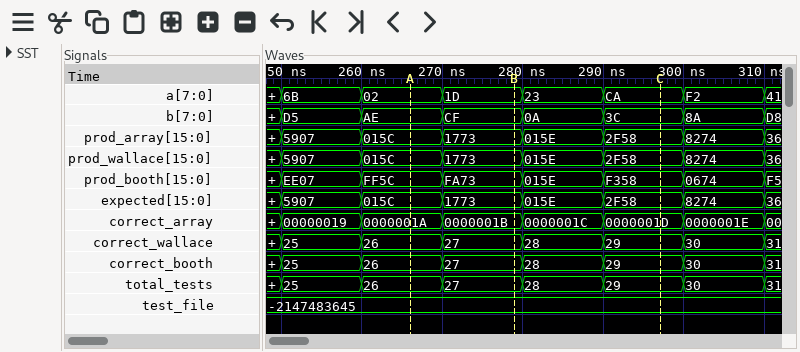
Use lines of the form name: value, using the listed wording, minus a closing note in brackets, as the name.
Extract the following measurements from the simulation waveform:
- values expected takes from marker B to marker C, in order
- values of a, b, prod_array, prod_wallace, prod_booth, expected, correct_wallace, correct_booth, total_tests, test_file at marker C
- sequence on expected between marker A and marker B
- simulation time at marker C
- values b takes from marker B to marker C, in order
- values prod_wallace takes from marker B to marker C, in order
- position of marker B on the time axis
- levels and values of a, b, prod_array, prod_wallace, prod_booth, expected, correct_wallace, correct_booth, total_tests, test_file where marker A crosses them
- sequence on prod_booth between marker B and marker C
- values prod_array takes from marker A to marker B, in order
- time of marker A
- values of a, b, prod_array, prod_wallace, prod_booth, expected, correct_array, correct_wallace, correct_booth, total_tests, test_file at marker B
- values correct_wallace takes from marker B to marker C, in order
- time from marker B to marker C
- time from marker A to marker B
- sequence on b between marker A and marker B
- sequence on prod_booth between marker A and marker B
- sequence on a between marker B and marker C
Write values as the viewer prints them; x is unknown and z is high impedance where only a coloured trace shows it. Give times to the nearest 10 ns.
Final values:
values expected takes from marker B to marker C, in order: 1773, 015E, 2F58
values of a, b, prod_array, prod_wallace, prod_booth, expected, correct_wallace, correct_booth, total_tests, test_file at marker C: a=CA, b=3C, prod_array=2F58, prod_wallace=2F58, prod_booth=F358, expected=2F58, correct_wallace=29, correct_booth=29, total_tests=29, test_file=-2147483645
sequence on expected between marker A and marker B: 015C, 1773
simulation time at marker C: 300 ns
values b takes from marker B to marker C, in order: CF, 0A, 3C
values prod_wallace takes from marker B to marker C, in order: 1773, 015E, 2F58
position of marker B on the time axis: 280 ns
levels and values of a, b, prod_array, prod_wallace, prod_booth, expected, correct_wallace, correct_booth, total_tests, test_file where marker A crosses them: a=02, b=AE, prod_array=015C, prod_wallace=015C, prod_booth=FF5C, expected=015C, correct_wallace=26, correct_booth=26, total_tests=26, test_file=-2147483645
sequence on prod_booth between marker B and marker C: FA73, 015E, F358
values prod_array takes from marker A to marker B, in order: 015C, 1773
time of marker A: 270 ns
values of a, b, prod_array, prod_wallace, prod_booth, expected, correct_array, correct_wallace, correct_booth, total_tests, test_file at marker B: a=1D, b=CF, prod_array=1773, prod_wallace=1773, prod_booth=FA73, expected=1773, correct_array=0000001B, correct_wallace=27, correct_booth=27, total_tests=27, test_file=-2147483645
values correct_wallace takes from marker B to marker C, in order: 27, 28, 29
time from marker B to marker C: 20 ns
time from marker A to marker B: 10 ns
sequence on b between marker A and marker B: AE, CF
sequence on prod_booth between marker A and marker B: FF5C, FA73
sequence on a between marker B and marker C: 1D, 23, CA
